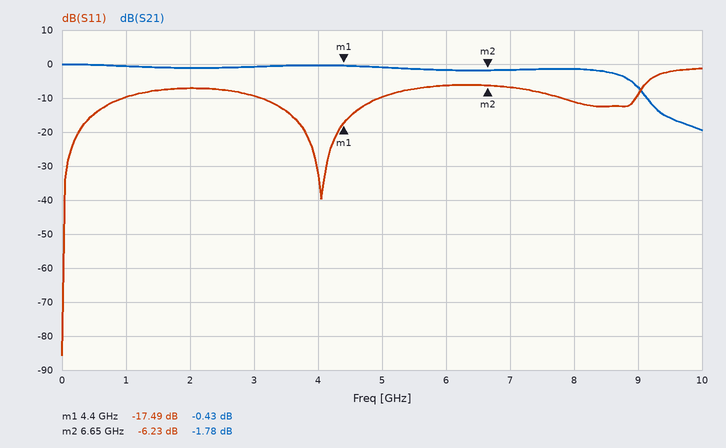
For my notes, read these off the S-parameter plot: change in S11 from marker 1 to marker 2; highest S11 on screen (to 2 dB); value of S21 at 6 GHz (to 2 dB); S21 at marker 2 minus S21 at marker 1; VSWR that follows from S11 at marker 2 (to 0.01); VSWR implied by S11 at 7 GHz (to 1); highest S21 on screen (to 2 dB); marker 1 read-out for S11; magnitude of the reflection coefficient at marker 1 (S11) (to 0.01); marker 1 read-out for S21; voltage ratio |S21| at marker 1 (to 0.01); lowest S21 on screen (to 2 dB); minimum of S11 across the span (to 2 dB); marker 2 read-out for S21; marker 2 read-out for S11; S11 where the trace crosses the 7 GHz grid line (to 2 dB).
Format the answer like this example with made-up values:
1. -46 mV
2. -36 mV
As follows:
1. 11.26 dB
2. -2 dB
3. -2 dB
4. -1.35 dB
5. 2.91
6. 3
7. 0 dB
8. -17.49 dB
9. 0.13
10. -0.43 dB
11. 0.95
12. -20 dB
13. -86 dB
14. -1.78 dB
15. -6.23 dB
16. -6 dB
